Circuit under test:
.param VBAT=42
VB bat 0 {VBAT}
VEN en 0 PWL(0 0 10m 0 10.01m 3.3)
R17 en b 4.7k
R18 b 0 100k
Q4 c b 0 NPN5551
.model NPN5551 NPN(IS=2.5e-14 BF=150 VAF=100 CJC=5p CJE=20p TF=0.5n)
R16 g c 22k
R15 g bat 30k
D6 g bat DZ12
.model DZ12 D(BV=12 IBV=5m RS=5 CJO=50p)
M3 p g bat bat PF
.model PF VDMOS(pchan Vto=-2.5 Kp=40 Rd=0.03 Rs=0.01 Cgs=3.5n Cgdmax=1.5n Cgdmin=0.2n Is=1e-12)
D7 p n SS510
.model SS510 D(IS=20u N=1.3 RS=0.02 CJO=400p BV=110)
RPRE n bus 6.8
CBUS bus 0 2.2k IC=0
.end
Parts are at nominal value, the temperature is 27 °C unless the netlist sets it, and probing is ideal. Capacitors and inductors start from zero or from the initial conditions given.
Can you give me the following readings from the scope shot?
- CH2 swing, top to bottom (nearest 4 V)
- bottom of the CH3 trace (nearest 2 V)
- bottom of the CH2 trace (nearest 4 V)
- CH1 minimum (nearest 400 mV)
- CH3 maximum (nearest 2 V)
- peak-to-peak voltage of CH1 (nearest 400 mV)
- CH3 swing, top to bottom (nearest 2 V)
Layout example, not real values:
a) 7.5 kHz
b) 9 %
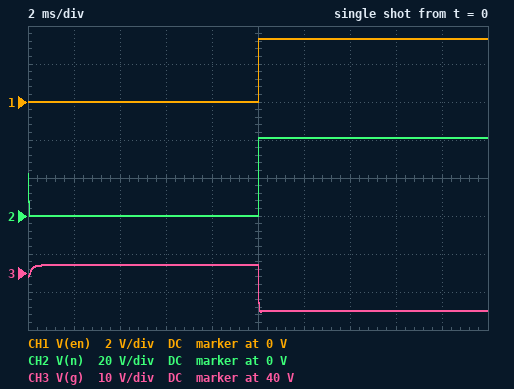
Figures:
a) 40 V
b) 30 V
c) 0 V
d) 0 V
e) 42 V
f) 3.2 V
g) 12 V
